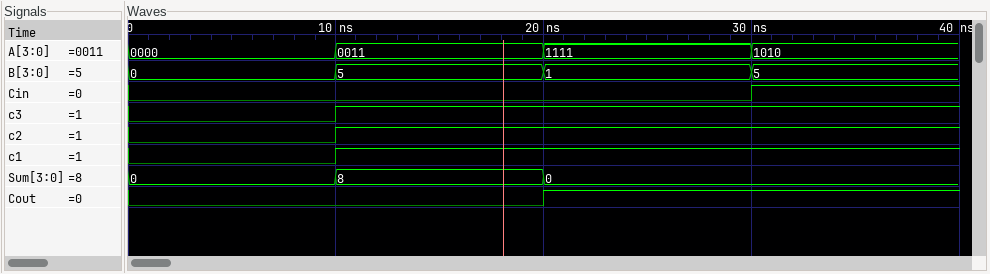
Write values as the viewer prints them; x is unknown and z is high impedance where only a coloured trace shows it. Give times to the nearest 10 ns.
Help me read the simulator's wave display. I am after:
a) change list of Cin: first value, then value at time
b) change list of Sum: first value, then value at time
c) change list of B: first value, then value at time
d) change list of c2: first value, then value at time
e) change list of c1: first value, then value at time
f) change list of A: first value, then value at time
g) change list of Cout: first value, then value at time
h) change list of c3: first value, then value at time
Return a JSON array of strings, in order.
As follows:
["0, 1 at 30 ns", "0, 8 at 10 ns, 0 at 20 ns", "0, 5 at 10 ns, 1 at 20 ns, 5 at 30 ns", "0, 1 at 10 ns", "0, 1 at 10 ns", "0000, 0011 at 10 ns, 1111 at 20 ns, 1010 at 30 ns", "0, 1 at 20 ns", "0, 1 at 10 ns"]
